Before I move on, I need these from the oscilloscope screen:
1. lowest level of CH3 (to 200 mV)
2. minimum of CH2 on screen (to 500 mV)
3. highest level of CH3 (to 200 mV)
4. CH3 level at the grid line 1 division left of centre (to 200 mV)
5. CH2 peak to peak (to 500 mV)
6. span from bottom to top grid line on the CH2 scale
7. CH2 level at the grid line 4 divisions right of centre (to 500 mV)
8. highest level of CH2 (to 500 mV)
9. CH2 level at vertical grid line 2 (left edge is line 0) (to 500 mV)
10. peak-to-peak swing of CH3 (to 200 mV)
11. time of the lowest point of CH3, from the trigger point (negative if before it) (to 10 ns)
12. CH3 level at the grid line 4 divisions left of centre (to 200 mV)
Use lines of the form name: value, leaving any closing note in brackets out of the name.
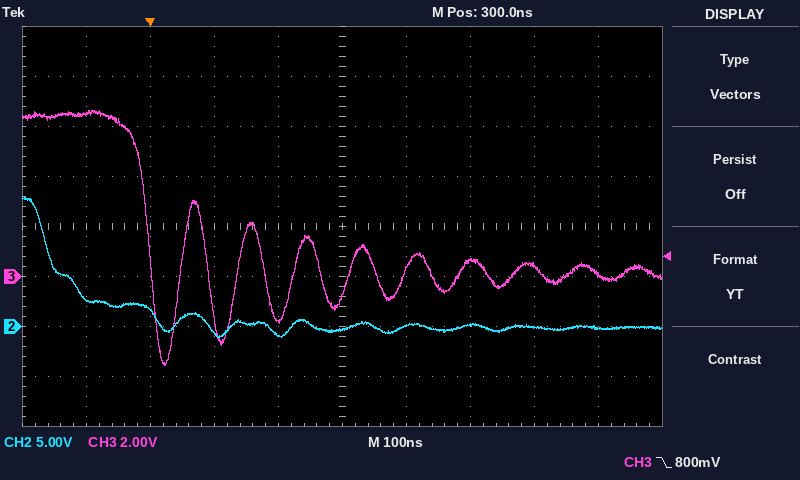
lowest level of CH3: -3.6 V
minimum of CH2 on screen: -1.0 V
highest level of CH3: 6.6 V
CH3 level at the grid line 1 division left of centre: -1.8 V
CH2 peak to peak: 14.0 V
span from bottom to top grid line on the CH2 scale: 40 V
CH2 level at the grid line 4 divisions right of centre: 0.0 V
highest level of CH2: 13.0 V
CH2 level at vertical grid line 2 (left edge is line 0): 1.5 V
peak-to-peak swing of CH3: 10.2 V
time of the lowest point of CH3, from the trigger point (negative if before it): +20 ns
CH3 level at the grid line 4 divisions left of centre: 6.6 V
